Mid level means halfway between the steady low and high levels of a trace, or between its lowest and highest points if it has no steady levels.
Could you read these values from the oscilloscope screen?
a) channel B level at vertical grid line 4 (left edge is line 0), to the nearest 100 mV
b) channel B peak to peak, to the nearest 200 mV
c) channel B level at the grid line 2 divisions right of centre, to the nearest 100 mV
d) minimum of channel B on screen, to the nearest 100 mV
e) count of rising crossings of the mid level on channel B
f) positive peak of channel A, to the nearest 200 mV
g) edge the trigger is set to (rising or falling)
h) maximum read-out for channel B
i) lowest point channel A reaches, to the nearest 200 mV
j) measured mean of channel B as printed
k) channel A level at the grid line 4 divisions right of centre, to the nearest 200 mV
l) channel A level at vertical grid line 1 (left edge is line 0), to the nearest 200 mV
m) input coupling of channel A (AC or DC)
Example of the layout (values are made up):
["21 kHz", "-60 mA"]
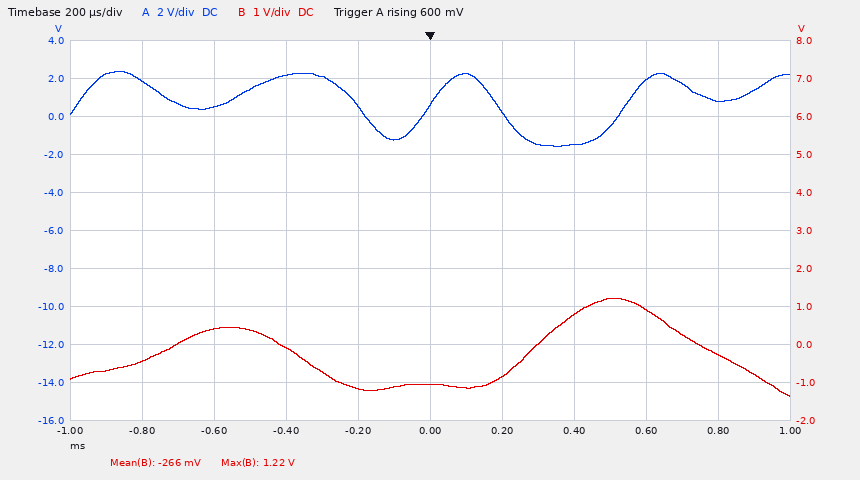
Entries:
["-1.2 V", "2.6 V", "800 mV", "-1.4 V", "2", "2.4 V", "rising", "1.22 V", "-1.6 V", "-266 mV", "800 mV", "1.8 V", "DC"]
